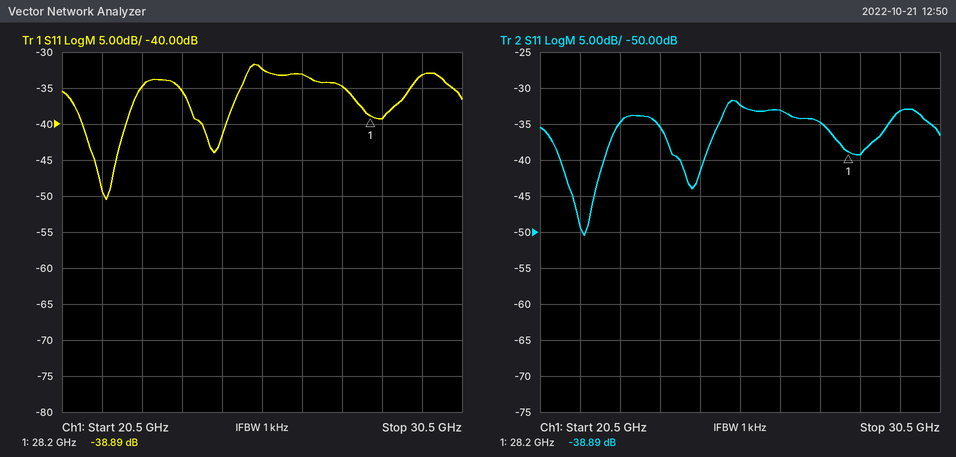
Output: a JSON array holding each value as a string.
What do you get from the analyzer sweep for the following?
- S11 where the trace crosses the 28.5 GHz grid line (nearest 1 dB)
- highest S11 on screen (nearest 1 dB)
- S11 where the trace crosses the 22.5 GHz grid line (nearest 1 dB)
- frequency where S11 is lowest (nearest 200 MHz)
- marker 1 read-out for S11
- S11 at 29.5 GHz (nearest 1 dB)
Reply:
["-39 dB", "-32 dB", "-35 dB", "21.6 GHz", "-38.89 dB", "-33 dB"]
